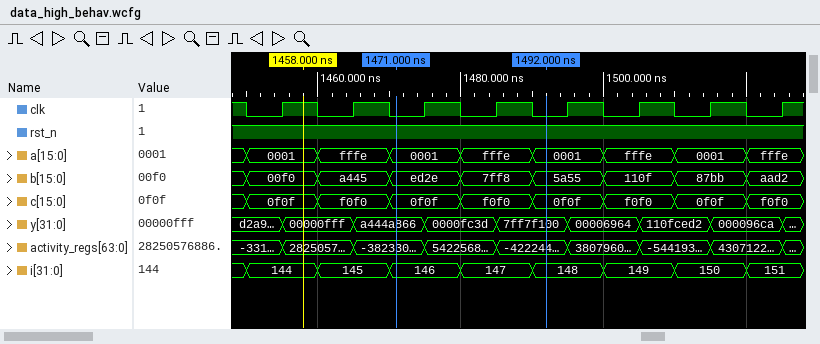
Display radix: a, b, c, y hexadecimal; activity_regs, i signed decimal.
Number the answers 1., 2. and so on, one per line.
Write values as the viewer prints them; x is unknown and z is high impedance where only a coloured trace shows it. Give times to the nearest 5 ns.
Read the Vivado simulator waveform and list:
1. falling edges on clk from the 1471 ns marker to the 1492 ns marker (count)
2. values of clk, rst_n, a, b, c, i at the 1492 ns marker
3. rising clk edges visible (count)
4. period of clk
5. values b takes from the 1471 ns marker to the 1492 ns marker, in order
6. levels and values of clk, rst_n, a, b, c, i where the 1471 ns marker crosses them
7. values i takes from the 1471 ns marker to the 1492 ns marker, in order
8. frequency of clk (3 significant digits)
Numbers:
1. 2
2. clk=0, rst_n=1, a=0001, b=5a55, c=0f0f, i=148
3. 8
4. 10 ns
5. ed2e, 7ff8, 5a55
6. clk=0, rst_n=1, a=0001, b=ed2e, c=0f0f, i=146
7. 146, 147, 148
8. 100 MHz
